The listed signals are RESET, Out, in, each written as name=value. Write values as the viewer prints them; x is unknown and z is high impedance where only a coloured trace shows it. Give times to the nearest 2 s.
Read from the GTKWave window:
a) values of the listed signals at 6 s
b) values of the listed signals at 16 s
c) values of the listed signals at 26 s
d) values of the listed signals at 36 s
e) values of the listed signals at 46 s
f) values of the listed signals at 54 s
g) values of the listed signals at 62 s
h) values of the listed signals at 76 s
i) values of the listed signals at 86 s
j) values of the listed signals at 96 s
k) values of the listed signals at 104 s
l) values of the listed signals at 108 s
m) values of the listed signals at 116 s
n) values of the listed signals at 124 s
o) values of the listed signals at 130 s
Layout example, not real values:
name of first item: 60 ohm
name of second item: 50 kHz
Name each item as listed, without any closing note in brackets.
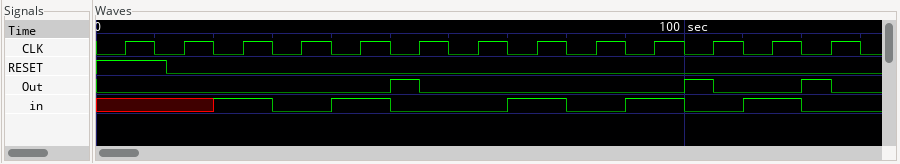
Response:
values of the listed signals at 6 s: RESET=1, Out=0, in=x
values of the listed signals at 16 s: RESET=0, Out=0, in=x
values of the listed signals at 26 s: RESET=0, Out=0, in=1
values of the listed signals at 36 s: RESET=0, Out=0, in=0
values of the listed signals at 46 s: RESET=0, Out=0, in=1
values of the listed signals at 54 s: RESET=0, Out=1, in=0
values of the listed signals at 62 s: RESET=0, Out=0, in=0
values of the listed signals at 76 s: RESET=0, Out=0, in=1
values of the listed signals at 86 s: RESET=0, Out=0, in=0
values of the listed signals at 96 s: RESET=0, Out=0, in=1
values of the listed signals at 104 s: RESET=0, Out=1, in=0
values of the listed signals at 108 s: RESET=0, Out=0, in=0
values of the listed signals at 116 s: RESET=0, Out=0, in=1
values of the listed signals at 124 s: RESET=0, Out=1, in=0
values of the listed signals at 130 s: RESET=0, Out=0, in=0
